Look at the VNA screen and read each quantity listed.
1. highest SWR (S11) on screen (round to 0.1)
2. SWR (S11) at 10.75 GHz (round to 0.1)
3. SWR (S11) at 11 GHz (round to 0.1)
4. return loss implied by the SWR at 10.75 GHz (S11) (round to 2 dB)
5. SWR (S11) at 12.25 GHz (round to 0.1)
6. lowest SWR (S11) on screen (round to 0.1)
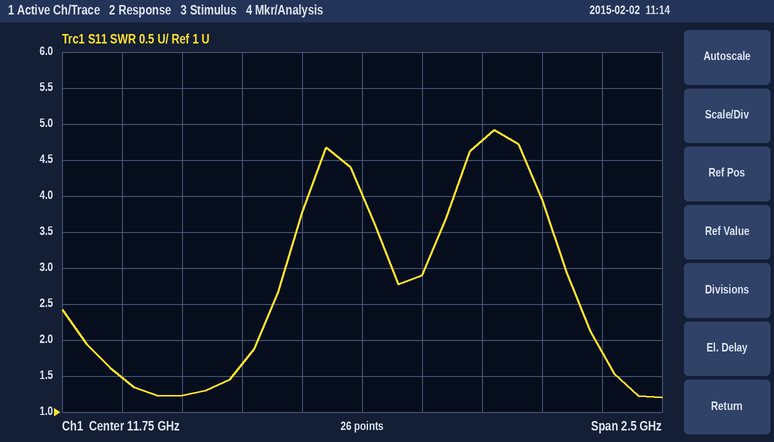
4.9
1.5
1.2
14 dB
4.8
1.2
